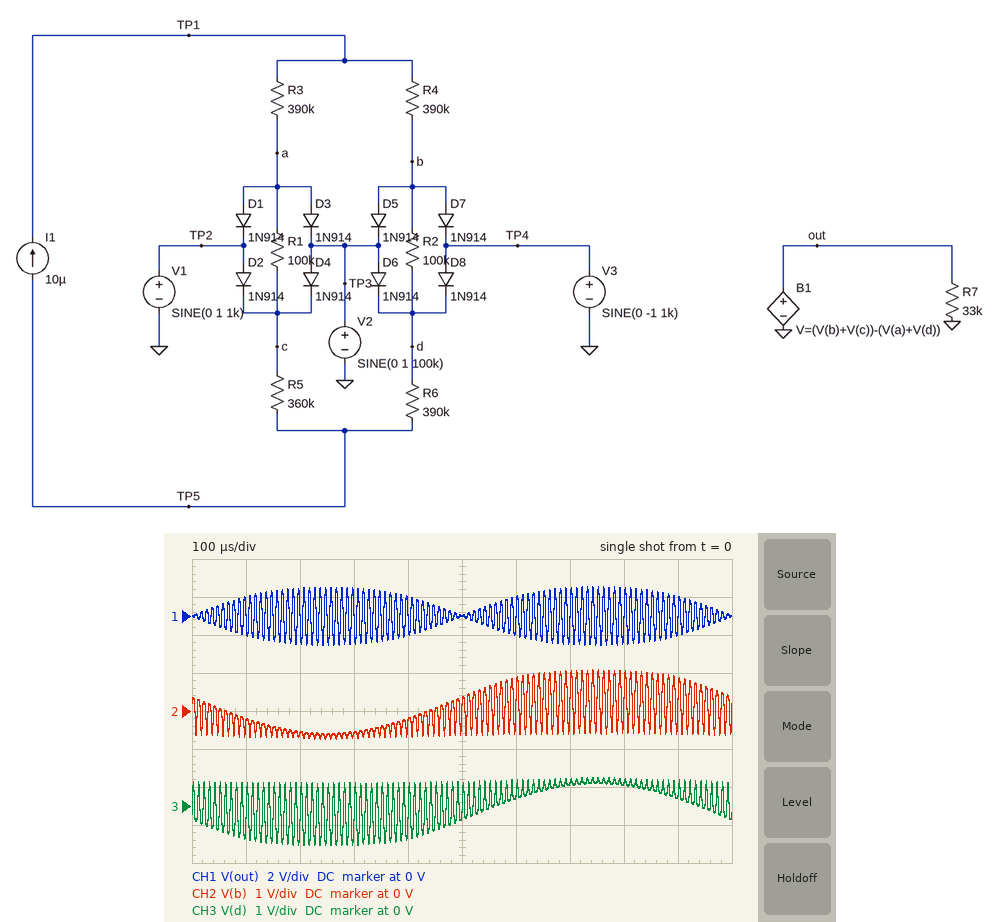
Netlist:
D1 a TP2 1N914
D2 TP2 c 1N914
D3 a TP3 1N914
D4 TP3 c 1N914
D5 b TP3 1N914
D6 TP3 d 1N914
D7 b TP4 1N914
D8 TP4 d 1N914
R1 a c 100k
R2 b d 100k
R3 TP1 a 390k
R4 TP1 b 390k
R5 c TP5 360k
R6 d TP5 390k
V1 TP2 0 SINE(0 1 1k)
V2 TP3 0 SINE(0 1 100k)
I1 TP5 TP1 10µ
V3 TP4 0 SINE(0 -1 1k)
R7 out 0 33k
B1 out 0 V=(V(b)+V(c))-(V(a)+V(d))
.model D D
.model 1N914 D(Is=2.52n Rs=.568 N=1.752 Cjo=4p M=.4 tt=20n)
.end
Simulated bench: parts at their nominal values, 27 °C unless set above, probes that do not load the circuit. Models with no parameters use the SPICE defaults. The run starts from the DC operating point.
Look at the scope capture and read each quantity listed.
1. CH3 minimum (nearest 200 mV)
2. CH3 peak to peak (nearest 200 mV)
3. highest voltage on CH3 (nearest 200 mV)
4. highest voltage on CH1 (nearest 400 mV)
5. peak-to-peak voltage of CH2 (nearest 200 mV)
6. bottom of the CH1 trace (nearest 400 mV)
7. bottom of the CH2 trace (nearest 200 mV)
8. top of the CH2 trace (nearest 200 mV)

-1.0 V
1.8 V
800 mV
1.6 V
1.8 V
-1.6 V
-800 mV
1.0 V
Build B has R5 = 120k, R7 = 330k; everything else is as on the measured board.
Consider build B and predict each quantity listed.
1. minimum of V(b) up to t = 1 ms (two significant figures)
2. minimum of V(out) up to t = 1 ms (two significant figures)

-690 mV
-1.6 V
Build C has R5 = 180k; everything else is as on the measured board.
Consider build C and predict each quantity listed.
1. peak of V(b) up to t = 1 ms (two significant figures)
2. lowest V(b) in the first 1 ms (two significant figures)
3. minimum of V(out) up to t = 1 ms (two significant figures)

1.1 V
-700 mV
-1.6 V
